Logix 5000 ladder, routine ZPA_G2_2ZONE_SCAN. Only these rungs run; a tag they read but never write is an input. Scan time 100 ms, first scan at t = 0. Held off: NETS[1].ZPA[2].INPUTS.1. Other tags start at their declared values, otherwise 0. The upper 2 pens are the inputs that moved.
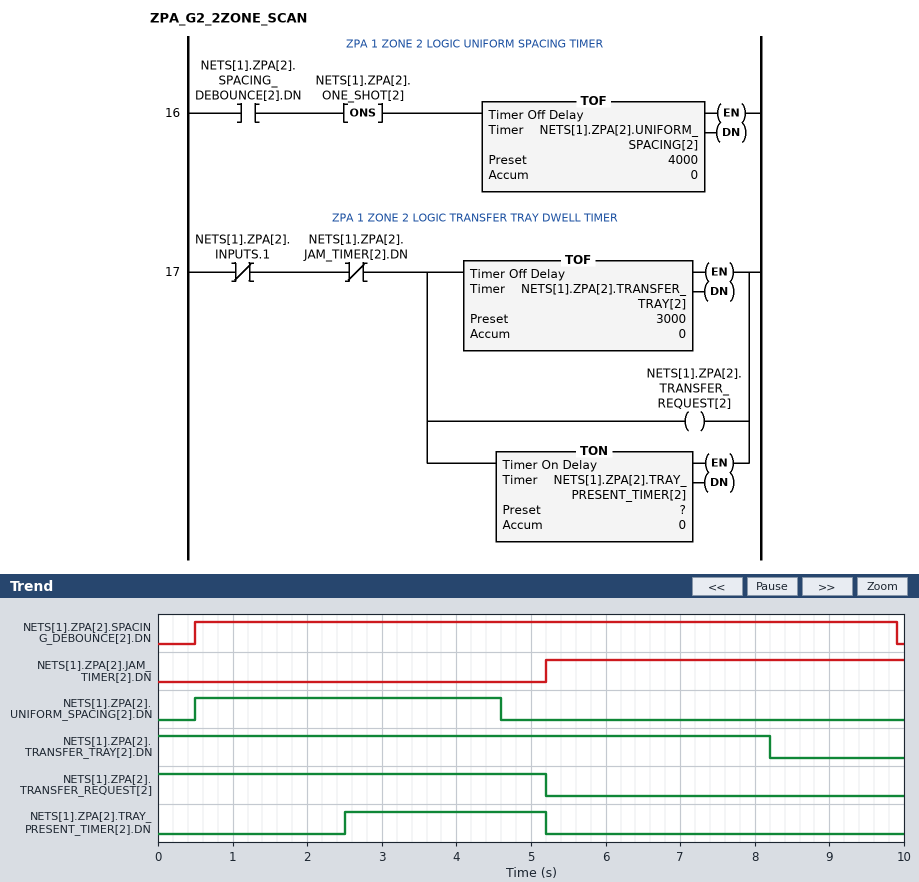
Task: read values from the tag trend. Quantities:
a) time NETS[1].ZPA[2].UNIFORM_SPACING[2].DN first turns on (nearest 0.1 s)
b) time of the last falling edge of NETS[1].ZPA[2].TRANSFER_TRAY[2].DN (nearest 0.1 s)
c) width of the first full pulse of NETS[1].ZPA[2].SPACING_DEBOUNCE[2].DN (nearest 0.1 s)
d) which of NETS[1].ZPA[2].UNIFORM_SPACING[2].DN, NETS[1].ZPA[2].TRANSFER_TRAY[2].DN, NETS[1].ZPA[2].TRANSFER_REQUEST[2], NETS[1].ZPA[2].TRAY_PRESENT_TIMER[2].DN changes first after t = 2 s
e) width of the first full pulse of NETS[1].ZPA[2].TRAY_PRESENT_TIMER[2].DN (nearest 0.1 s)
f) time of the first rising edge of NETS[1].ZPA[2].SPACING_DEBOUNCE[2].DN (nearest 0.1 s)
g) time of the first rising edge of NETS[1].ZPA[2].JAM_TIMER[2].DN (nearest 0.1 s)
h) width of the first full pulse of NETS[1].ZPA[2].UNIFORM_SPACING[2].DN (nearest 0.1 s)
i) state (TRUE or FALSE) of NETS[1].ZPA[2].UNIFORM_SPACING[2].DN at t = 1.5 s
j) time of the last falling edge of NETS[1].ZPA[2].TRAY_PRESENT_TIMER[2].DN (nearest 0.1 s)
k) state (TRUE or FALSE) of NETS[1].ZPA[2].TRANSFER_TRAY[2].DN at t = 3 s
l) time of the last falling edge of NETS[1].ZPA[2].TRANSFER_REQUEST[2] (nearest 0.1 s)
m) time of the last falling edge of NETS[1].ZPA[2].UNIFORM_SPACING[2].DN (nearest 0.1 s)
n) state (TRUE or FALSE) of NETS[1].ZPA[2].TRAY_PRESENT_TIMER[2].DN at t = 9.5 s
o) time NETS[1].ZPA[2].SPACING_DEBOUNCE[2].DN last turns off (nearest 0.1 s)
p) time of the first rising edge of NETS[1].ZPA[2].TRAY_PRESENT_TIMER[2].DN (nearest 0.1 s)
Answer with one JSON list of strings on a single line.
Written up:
["0.5 s", "8.2 s", "9.4 s", "NETS[1].ZPA[2].TRAY_PRESENT_TIMER[2].DN", "2.7 s", "0.5 s", "5.2 s", "4.1 s", "TRUE", "5.2 s", "TRUE", "5.2 s", "4.6 s", "FALSE", "9.9 s", "2.5 s"]
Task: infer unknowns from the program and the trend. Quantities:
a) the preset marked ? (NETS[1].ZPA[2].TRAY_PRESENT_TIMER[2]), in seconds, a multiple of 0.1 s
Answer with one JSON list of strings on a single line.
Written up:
["2.5 s"]
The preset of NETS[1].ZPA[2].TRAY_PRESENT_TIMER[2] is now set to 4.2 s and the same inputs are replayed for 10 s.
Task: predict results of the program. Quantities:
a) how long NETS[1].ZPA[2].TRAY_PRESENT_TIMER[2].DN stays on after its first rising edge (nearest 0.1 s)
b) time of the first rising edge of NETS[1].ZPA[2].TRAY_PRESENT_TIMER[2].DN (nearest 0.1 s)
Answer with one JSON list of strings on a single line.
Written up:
["1.0 s", "4.2 s"]
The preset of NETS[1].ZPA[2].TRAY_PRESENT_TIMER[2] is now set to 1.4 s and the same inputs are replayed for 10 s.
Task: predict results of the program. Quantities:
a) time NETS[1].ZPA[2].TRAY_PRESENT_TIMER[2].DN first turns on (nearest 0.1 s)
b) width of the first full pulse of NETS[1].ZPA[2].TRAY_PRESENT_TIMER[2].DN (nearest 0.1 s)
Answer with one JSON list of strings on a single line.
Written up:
["1.4 s", "3.8 s"]
